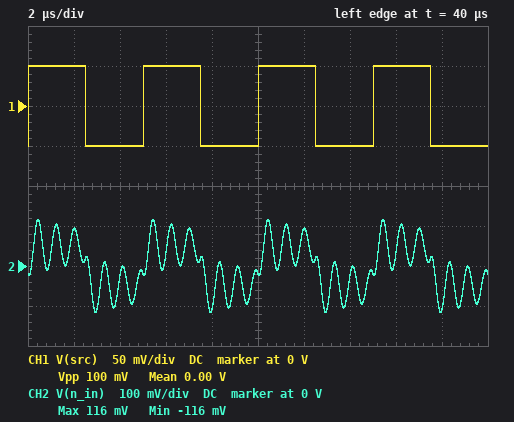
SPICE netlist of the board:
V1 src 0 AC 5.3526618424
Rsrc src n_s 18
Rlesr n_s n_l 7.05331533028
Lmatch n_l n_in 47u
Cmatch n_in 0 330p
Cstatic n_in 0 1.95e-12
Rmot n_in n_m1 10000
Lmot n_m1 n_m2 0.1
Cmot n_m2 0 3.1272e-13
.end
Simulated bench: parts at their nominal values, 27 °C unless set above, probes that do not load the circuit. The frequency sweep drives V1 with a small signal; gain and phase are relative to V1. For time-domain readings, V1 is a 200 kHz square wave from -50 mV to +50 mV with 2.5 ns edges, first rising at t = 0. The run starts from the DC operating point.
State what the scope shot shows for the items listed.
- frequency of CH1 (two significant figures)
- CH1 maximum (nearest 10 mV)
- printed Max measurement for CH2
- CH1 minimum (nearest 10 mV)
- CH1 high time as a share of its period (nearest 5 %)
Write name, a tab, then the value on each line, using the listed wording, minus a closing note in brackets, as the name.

frequency of CH1	200 kHz
CH1 maximum	50 mV
printed Max measurement for CH2	116 mV
CH1 minimum	-50 mV
CH1 high time as a share of its period	50 %
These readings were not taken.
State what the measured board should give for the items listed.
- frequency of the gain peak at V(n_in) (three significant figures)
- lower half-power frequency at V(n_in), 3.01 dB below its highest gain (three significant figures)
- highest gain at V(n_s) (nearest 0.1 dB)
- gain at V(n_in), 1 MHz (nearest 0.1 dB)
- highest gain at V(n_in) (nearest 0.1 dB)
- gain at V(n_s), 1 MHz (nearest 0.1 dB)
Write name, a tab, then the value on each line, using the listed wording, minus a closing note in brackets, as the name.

frequency of the gain peak at V(n_in)	1.27 MHz
lower half-power frequency at V(n_in), 3.01 dB below its highest gain	1.23 MHz
highest gain at V(n_s)	0 dB
gain at V(n_in), 1 MHz	8.2 dB
highest gain at V(n_in)	23.5 dB
gain at V(n_s), 1 MHz	-0.1 dB
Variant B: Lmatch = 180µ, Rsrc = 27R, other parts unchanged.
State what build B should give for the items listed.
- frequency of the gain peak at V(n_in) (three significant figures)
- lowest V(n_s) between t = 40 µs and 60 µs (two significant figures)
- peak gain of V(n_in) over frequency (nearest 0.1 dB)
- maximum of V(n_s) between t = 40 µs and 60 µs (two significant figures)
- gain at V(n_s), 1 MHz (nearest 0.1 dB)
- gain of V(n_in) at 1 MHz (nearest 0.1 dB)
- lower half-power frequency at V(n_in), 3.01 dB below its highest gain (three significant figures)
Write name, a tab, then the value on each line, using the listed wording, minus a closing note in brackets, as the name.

frequency of the gain peak at V(n_in)	650 kHz
lowest V(n_s) between t = 40 µs and 60 µs	-55 mV
peak gain of V(n_in) over frequency	26.7 dB
maximum of V(n_s) between t = 40 µs and 60 µs	55 mV
gain at V(n_s), 1 MHz	0 dB
gain of V(n_in) at 1 MHz	-2.6 dB
lower half-power frequency at V(n_in), 3.01 dB below its highest gain	635 kHz
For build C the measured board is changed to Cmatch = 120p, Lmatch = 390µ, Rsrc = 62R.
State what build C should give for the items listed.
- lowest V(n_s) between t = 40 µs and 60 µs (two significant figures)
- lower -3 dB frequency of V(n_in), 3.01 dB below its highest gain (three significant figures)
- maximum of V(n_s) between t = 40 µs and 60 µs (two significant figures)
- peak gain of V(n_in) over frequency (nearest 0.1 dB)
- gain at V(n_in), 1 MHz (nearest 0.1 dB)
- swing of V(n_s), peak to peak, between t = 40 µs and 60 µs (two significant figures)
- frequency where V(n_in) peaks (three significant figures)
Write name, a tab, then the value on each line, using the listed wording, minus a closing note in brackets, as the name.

lowest V(n_s) between t = 40 µs and 60 µs	-52 mV
lower -3 dB frequency of V(n_in), 3.01 dB below its highest gain	713 kHz
maximum of V(n_s) between t = 40 µs and 60 µs	52 mV
peak gain of V(n_in) over frequency	28.2 dB
gain at V(n_in), 1 MHz	1.3 dB
swing of V(n_s), peak to peak, between t = 40 µs and 60 µs	100 mV
frequency where V(n_in) peaks	727 kHz
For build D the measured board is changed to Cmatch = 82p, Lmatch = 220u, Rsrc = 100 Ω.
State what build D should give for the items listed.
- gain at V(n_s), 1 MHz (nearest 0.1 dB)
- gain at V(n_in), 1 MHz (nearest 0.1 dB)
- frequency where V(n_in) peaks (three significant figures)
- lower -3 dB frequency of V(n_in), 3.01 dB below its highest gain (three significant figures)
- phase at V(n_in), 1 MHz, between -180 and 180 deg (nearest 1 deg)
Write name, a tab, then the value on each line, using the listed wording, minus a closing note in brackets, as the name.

gain at V(n_s), 1 MHz	-0.2 dB
gain at V(n_in), 1 MHz	10.8 dB
frequency where V(n_in) peaks	1.17 MHz
lower -3 dB frequency of V(n_in), 3.01 dB below its highest gain	1.13 MHz
phase at V(n_in), 1 MHz, between -180 and 180 deg	-11 deg
